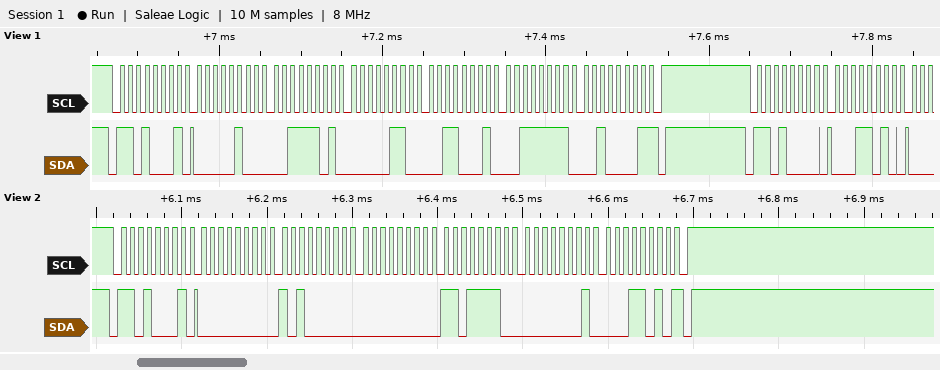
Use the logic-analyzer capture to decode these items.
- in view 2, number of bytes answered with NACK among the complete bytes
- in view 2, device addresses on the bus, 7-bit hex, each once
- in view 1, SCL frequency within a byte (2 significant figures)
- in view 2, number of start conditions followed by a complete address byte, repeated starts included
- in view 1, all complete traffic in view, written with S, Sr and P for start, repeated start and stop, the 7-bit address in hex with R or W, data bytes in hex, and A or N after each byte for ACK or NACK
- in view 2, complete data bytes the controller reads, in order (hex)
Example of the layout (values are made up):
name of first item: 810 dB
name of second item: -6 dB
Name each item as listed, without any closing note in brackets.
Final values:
in view 2, number of bytes answered with NACK among the complete bytes: 1
in view 2, device addresses on the bus, 7-bit hex, each once: 0x68
in view 1, SCL frequency within a byte: 100 kHz
in view 2, number of start conditions followed by a complete address byte, repeated starts included: 1
in view 1, all complete traffic in view, written with S, Sr and P for start, repeated start and stop, the 7-bit address in hex with R or W, data bytes in hex, and A or N after each byte for ACK or NACK: S 68R A 04 A 3D A 06 A 31 A 3F A 21 N P S 68W A 1A A
in view 2, complete data bytes the controller reads, in order: 00 A0 00 DE 01 1A
